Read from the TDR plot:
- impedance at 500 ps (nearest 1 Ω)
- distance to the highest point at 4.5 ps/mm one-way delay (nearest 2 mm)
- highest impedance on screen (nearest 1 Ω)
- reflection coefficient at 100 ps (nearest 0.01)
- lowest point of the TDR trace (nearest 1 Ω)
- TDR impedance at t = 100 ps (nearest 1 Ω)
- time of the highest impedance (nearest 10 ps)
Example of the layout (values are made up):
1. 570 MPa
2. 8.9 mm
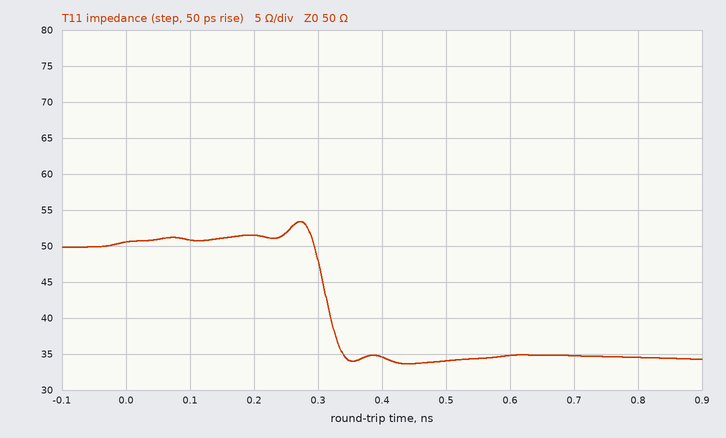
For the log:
1. 34 Ω
2. 30 mm
3. 53 Ω
4. +0.01
5. 34 Ω
6. 51 Ω
7. 270 ps
